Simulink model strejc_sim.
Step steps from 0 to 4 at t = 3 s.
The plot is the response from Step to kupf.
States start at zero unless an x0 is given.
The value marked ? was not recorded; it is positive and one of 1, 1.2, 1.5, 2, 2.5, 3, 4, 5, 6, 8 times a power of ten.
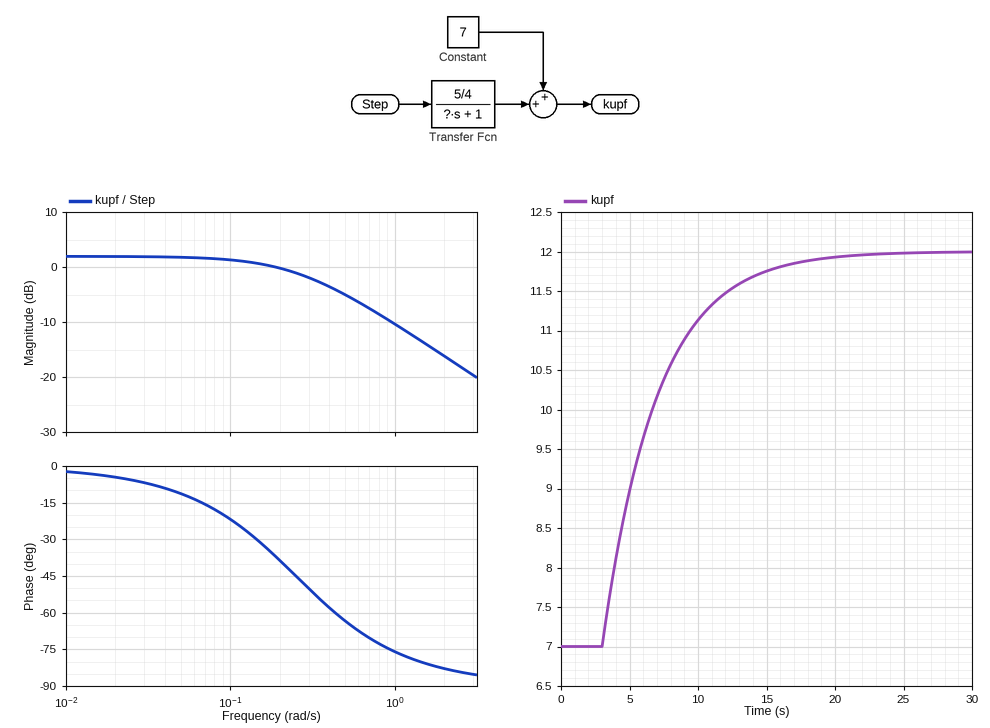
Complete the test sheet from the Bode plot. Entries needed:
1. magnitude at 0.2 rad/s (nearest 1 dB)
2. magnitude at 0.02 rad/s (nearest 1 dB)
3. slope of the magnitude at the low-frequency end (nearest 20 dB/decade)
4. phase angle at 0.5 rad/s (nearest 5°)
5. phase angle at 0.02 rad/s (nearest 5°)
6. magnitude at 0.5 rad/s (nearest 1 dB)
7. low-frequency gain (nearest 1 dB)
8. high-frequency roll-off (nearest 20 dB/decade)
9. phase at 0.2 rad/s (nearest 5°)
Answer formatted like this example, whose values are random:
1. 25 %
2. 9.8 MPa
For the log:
1. 0 dB
2. 2 dB
3. 0 dB/decade
4. -65°
5. -5°
6. -5 dB
7. 2 dB
8. -20 dB/decade
9. -40°
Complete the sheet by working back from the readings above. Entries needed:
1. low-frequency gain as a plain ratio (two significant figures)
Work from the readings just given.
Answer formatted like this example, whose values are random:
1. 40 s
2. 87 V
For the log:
1. 1.3
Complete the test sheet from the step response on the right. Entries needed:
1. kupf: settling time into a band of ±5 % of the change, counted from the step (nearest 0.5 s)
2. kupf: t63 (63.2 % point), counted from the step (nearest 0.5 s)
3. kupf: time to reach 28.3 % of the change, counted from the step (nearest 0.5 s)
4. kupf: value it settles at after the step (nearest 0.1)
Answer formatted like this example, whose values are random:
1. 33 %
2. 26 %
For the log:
1. 12.0 s
2. 4.0 s
3. 1.5 s
4. 12.0
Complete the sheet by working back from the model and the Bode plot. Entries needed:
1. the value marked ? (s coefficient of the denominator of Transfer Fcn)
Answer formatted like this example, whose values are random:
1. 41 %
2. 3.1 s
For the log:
1. 4
